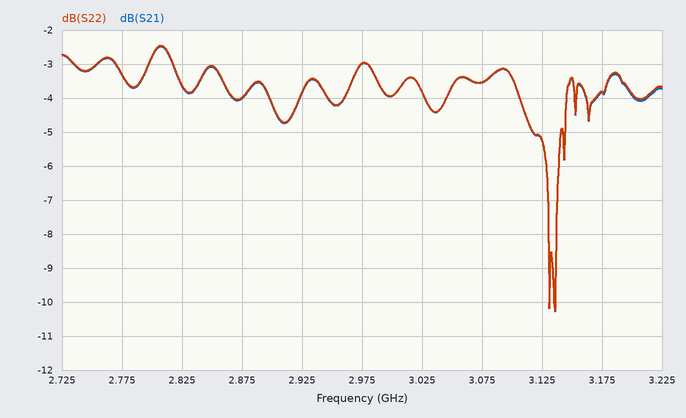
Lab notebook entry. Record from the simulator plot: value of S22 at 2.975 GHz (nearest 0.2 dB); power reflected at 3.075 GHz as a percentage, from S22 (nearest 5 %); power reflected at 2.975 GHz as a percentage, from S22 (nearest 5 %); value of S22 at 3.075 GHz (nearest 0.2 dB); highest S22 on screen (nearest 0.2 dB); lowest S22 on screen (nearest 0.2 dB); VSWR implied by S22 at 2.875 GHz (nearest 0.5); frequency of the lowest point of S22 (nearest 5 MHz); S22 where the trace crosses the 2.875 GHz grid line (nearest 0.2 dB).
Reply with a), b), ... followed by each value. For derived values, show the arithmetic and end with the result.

a) -3.0 dB
b) 10^(-3.6/10) ≈ 43.7 %, so 45 % to the nearest 5 %
c) 10^(-3/10) ≈ 50 %
d) -3.6 dB
e) -2.4 dB
f) -10.2 dB
g) |Γ| = 10^(-4/20) = 0.6310; VSWR = (1 + 0.6310)/(1 − 0.6310) ≈ 4.42, so 4.5 to the nearest 0.5
h) 3.135 GHz
i) -4.0 dB
